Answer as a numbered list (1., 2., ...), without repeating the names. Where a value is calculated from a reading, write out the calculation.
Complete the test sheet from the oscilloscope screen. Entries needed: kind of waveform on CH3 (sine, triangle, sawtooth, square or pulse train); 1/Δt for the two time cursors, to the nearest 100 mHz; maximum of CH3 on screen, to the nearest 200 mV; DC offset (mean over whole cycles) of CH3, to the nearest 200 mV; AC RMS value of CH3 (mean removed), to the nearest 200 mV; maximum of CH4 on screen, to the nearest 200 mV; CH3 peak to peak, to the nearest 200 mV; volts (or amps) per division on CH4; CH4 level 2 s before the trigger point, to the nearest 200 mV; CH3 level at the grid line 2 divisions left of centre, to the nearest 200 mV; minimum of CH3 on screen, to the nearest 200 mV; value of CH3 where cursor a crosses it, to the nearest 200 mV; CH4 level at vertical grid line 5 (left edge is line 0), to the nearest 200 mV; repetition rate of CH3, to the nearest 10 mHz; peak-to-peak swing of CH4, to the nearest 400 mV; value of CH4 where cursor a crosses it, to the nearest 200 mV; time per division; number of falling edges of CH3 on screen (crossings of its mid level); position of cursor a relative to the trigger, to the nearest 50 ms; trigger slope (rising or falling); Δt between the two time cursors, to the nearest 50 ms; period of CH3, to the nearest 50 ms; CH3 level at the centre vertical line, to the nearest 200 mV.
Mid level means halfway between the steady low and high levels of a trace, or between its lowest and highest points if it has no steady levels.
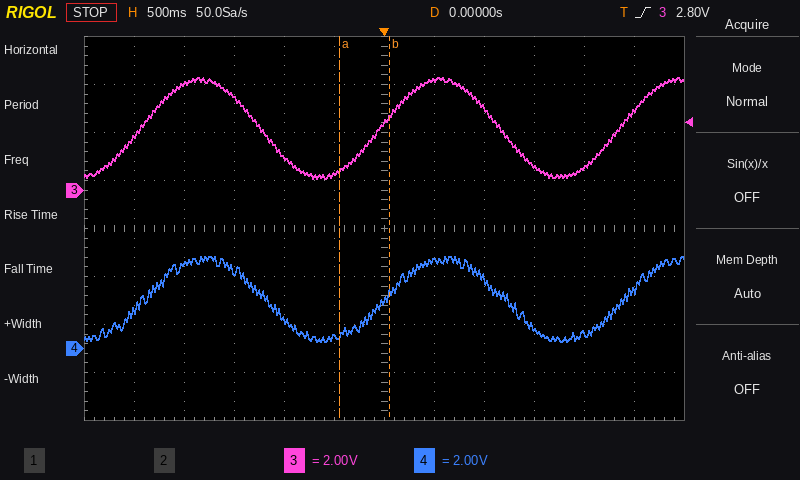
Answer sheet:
1. sine
2. 1 / 500 ms ≈ 2.0 Hz
3. 4.6 V
4. (4.6 V + (400 mV)) / 2 ≈ 2.50 V, so 2.6 V to the nearest 200 mV
5. 4.2 V / (2√2) ≈ 1.48 V, so 1.4 V to the nearest 200 mV
6. 3.8 V
7. 4.6 V − (400 mV) = 4.2 V
8. 2 V
9. 3.6 V
10. 1.4 V
11. 400 mV
12. 800 mV
13. 400 mV
14. 1 / 2.40 s ≈ 417 mHz, so 420 mHz to the nearest 10 mHz
15. 3.6 V
16. 600 mV
17. 500 ms
18. 2
19. -450 ms
20. rising
21. 500 ms
22. 2.40 s
23. 2.8 V
